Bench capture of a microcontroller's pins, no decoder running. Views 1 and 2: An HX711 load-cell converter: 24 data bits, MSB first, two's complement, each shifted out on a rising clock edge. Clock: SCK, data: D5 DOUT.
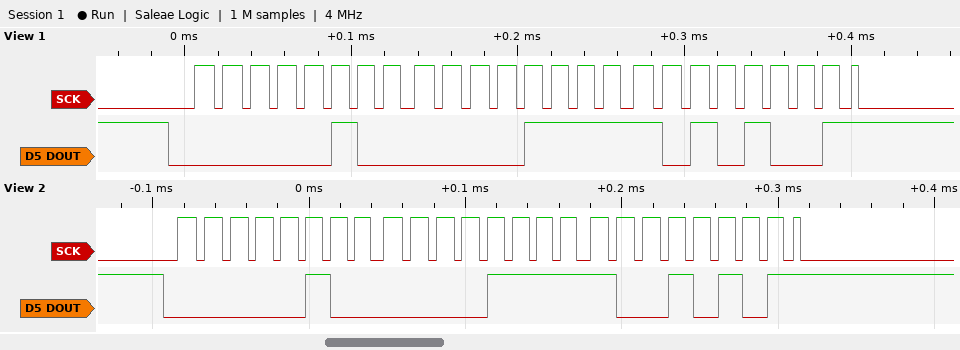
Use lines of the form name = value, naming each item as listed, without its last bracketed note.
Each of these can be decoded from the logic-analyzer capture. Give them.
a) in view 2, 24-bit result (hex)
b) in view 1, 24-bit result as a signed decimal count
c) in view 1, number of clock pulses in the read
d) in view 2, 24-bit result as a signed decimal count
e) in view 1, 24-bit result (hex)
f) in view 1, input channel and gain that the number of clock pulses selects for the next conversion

in view 2, 24-bit result = 0x040F95
in view 1, 24-bit result as a signed decimal count = 266153
in view 1, number of clock pulses in the read = 25
in view 2, 24-bit result as a signed decimal count = 266133
in view 1, 24-bit result = 0x040FA9
in view 1, input channel and gain that the number of clock pulses selects for the next conversion = channel A, gain 128
